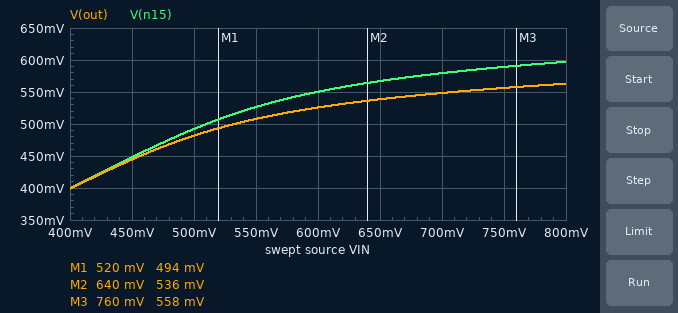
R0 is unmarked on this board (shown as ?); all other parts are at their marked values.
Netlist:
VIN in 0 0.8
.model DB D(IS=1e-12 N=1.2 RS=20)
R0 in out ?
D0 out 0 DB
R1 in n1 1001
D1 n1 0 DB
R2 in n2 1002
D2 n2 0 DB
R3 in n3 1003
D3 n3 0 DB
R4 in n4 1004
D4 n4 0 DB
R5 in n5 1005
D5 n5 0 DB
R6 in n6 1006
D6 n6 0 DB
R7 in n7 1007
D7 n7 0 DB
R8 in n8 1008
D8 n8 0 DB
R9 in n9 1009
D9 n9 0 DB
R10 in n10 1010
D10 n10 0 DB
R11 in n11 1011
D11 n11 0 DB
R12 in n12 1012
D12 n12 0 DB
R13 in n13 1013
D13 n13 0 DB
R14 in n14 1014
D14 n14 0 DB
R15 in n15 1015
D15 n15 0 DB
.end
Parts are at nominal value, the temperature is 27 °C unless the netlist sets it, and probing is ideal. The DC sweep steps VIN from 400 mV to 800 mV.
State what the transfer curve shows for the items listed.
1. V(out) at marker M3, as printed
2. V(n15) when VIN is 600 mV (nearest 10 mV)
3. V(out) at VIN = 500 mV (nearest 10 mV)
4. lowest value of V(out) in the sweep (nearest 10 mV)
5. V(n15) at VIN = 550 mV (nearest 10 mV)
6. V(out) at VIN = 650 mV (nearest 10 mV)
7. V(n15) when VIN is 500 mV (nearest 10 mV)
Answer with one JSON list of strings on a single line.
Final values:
["558 mV", "550 mV", "480 mV", "400 mV", "530 mV", "540 mV", "490 mV"]
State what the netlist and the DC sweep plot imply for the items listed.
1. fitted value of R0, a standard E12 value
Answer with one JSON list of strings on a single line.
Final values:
["3.3 kΩ"]
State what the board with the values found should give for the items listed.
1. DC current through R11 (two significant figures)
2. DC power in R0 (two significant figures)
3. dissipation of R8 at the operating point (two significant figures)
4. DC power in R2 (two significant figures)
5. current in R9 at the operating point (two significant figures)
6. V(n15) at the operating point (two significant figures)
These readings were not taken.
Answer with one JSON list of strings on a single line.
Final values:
["200 µA", "17 µW", "41 µW", "41 µW", "200 µA", "600 mV"]
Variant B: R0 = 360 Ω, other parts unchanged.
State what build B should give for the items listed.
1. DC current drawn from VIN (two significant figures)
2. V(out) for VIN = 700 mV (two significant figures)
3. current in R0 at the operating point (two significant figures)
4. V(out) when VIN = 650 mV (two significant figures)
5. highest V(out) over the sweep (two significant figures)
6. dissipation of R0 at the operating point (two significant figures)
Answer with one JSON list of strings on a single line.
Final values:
["3.5 mA", "610 mV", "470 µA", "590 mV", "630 mV", "81 µW"]
